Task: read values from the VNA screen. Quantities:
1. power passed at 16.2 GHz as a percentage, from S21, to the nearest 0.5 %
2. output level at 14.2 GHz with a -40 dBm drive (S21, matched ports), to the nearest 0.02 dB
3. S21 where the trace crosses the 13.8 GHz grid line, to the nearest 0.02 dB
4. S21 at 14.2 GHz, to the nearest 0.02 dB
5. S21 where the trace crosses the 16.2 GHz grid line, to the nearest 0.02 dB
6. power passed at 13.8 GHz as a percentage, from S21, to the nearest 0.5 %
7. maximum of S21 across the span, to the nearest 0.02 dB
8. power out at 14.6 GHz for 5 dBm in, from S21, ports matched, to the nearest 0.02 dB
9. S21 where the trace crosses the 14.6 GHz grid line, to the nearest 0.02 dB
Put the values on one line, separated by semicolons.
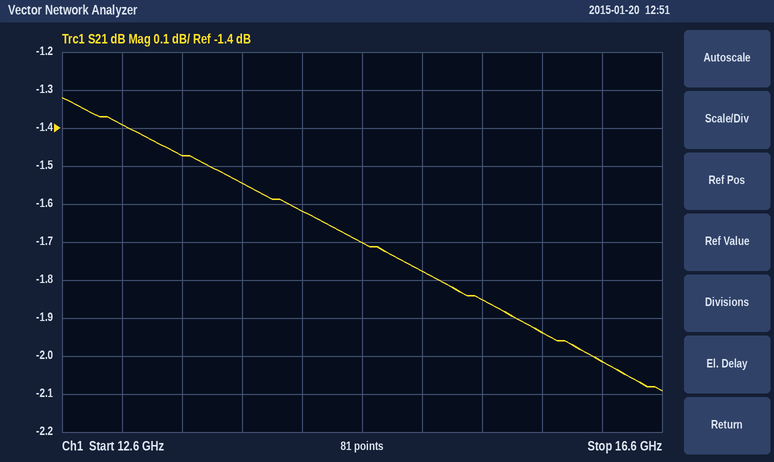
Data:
63.0 %; -41.62 dBm; -1.54 dB; -1.62 dB; -2.02 dB; 70.0 %; -1.32 dB; 3.30 dBm; -1.70 dB
